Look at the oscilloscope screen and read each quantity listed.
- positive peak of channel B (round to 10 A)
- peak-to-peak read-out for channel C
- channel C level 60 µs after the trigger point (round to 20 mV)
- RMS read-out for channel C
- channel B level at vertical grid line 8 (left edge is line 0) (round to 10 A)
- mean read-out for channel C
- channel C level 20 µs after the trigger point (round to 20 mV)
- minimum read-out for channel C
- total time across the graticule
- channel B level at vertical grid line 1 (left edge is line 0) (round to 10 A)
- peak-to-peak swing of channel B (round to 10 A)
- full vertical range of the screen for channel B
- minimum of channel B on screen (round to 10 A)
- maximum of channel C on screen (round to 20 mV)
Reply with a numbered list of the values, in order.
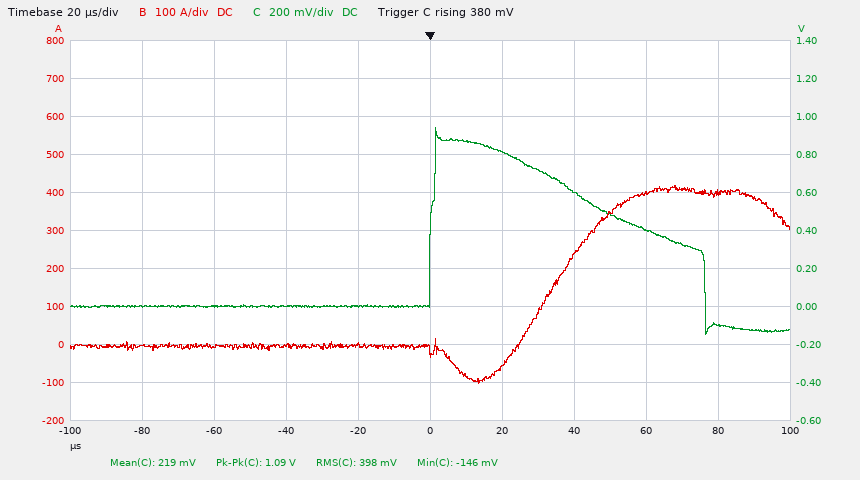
1. 420 A
2. 1.09 V
3. 400 mV
4. 398 mV
5. 400 A
6. 219 mV
7. 820 mV
8. -146 mV
9. 200 µs
10. 0 A
11. 520 A
12. 1 kA
13. -100 A
14. 940 mV
